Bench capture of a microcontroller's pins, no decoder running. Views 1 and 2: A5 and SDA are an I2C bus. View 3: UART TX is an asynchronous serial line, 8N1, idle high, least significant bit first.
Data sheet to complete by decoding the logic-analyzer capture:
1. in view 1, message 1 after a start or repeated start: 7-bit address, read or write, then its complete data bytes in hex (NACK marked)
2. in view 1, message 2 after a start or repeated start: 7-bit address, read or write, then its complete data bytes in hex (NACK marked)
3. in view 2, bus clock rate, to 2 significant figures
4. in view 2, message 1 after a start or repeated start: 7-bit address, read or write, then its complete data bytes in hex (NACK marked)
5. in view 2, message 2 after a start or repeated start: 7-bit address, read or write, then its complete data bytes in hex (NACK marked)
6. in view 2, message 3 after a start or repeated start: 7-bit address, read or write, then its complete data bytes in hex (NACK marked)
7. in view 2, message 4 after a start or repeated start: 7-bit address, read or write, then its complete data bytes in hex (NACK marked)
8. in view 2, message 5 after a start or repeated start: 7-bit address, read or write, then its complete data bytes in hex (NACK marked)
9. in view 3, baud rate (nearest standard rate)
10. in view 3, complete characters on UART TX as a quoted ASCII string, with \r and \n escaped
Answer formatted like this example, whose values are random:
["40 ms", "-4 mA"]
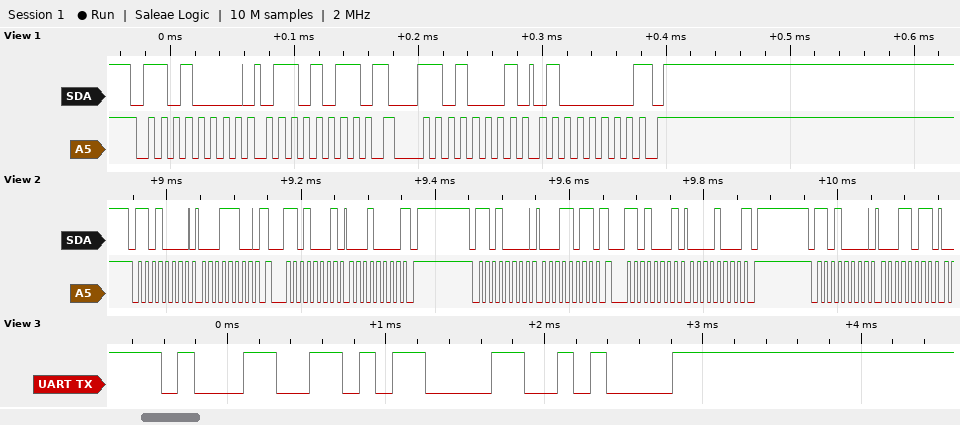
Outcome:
["0x68 write: 6B", "0x68 read: 40 NACK", "100 kHz", "0x68 write: 1C", "0x68 read: 10 NACK", "0x68 write: 1B", "0x68 read: 08 NACK", "0x68 write: 1B", "9600 baud", "\"1\\r\\n\""]
